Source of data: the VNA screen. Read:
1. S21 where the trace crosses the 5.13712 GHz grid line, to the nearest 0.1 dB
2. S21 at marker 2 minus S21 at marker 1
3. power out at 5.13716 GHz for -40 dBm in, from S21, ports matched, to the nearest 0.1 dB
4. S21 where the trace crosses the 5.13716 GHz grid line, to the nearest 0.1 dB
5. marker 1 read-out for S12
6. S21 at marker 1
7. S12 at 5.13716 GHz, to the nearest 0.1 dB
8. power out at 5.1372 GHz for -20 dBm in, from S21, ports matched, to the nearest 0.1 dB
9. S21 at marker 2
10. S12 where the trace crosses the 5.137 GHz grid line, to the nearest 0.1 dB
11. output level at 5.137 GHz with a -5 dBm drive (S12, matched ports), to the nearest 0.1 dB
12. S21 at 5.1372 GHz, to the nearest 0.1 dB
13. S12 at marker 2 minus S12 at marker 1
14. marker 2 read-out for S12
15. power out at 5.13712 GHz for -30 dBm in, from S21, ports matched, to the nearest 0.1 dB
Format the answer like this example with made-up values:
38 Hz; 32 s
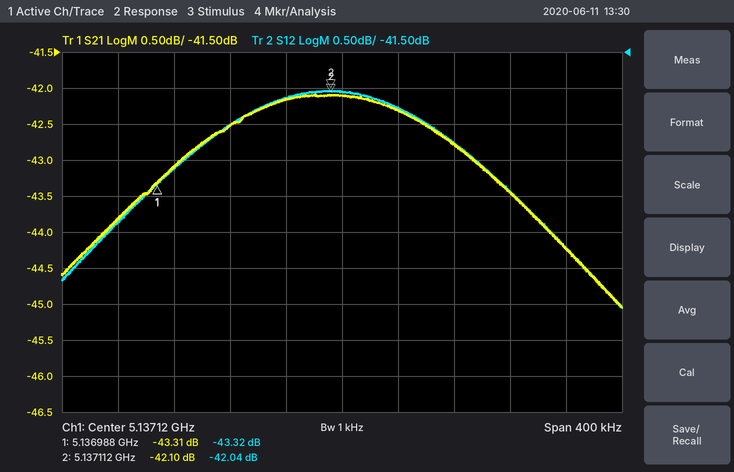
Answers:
-42.1 dB; 1.21 dB; -82.3 dBm; -42.3 dB; -43.32 dB; -43.31 dB; -42.3 dB; -62.8 dBm; -42.10 dB; -43.1 dB; -48.1 dBm; -42.8 dB; 1.28 dB; -42.04 dB; -72.1 dBm
